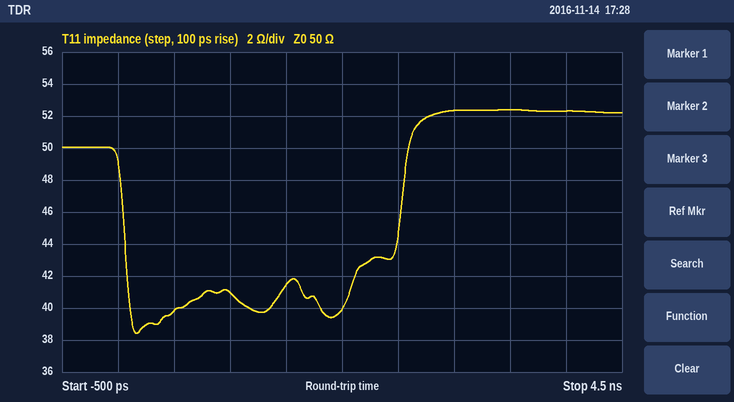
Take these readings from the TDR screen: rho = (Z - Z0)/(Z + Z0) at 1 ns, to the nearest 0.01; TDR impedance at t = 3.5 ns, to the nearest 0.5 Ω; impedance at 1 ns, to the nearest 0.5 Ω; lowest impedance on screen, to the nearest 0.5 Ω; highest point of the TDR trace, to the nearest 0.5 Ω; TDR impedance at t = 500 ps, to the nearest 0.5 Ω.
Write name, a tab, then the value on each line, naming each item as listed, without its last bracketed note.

rho = (Z - Z0)/(Z + Z0) at 1 ns, to the nearest 0.01	-0.10
TDR impedance at t = 3.5 ns, to the nearest 0.5 Ω	52.5 Ω
impedance at 1 ns, to the nearest 0.5 Ω	41.0 Ω
lowest impedance on screen, to the nearest 0.5 Ω	38.5 Ω
highest point of the TDR trace, to the nearest 0.5 Ω	52.5 Ω
TDR impedance at t = 500 ps, to the nearest 0.5 Ω	40.0 Ω
